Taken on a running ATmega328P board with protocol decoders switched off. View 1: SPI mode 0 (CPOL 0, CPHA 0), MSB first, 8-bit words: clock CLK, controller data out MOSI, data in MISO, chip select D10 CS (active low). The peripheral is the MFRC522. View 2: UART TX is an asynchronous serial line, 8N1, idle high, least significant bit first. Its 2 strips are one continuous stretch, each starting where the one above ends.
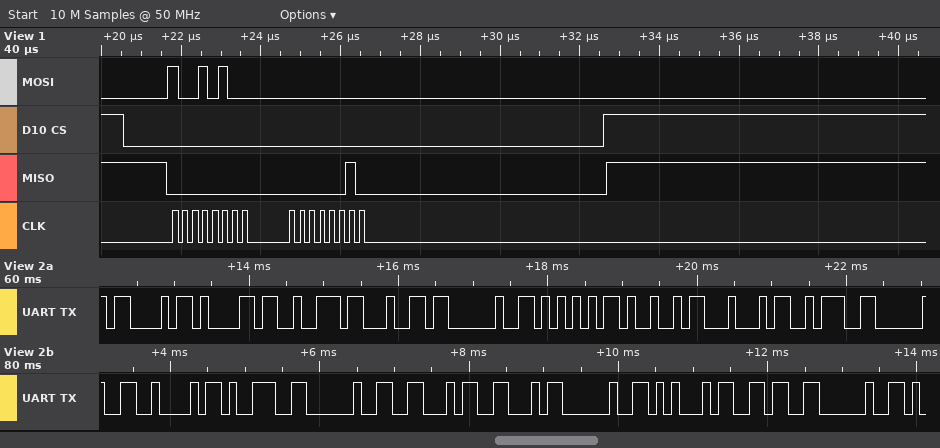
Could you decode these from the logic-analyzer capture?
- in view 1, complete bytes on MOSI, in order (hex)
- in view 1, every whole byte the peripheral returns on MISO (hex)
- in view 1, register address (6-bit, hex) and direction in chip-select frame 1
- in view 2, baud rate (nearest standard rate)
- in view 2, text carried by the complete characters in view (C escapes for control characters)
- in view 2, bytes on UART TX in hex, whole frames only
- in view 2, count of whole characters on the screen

94 00
00 02
0x0A read
9600 baud
"Card UID: B9 FF E6 "
43 61 72 64 20 55 49 44 3A 20 42 39 20 46 46 20 45 36 20
19
